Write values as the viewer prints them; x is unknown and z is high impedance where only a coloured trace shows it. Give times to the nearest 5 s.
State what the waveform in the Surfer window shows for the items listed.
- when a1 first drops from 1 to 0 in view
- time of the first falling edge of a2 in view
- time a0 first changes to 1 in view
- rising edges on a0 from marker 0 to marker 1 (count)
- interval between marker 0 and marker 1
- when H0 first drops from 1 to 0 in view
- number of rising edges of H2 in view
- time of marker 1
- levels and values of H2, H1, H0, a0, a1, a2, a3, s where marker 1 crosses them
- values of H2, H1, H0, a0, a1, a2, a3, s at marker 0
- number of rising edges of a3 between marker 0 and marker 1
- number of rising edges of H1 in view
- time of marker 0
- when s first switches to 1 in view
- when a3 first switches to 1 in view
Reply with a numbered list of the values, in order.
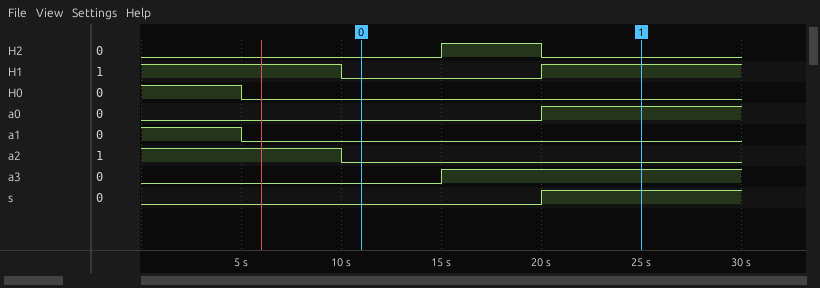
1. 5 s
2. 10 s
3. 20 s
4. 1
5. 15 s
6. 5 s
7. 1
8. 25 s
9. H2=0, H1=1, H0=0, a0=1, a1=0, a2=0, a3=1, s=1
10. H2=0, H1=0, H0=0, a0=0, a1=0, a2=0, a3=0, s=0
11. 1
12. 1
13. 10 s
14. 20 s
15. 15 s
